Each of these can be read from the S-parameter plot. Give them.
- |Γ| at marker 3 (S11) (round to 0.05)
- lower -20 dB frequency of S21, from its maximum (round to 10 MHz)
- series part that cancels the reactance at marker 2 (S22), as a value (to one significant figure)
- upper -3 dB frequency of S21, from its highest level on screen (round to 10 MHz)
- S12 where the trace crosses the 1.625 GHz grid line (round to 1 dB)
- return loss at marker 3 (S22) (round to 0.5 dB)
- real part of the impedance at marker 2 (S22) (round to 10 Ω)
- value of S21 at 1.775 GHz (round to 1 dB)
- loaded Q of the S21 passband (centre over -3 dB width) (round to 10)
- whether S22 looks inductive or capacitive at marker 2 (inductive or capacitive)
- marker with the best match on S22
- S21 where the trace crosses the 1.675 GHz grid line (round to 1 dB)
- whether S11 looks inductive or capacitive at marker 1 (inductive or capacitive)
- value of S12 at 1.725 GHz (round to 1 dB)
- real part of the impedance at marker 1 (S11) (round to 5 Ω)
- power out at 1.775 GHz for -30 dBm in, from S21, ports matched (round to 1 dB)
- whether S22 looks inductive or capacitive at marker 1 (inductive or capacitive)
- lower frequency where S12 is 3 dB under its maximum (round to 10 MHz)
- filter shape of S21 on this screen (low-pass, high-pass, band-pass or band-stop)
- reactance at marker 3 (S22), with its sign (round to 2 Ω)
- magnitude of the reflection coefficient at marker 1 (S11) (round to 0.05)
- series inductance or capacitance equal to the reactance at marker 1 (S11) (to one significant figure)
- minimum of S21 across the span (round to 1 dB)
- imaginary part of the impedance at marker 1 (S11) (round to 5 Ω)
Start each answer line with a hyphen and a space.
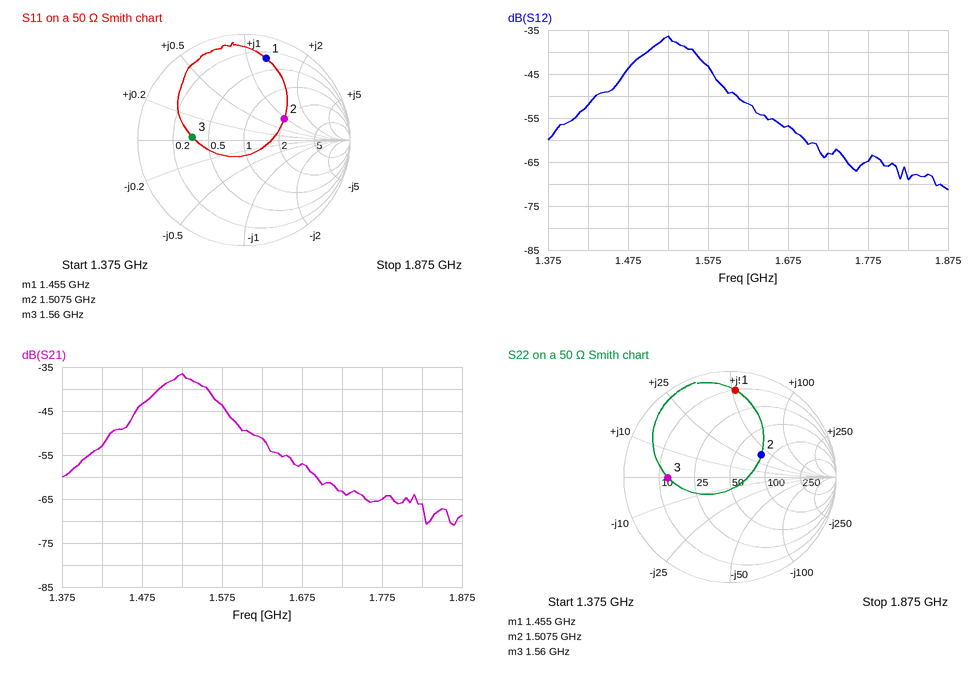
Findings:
- 0.50
- 1.40 GHz
- 3 pF
- 1.55 GHz
- -52 dB
- 4.5 dB
- 80 Ω
- -65 dB
- 30
- inductive
- marker 2
- -57 dB
- inductive
- -63 dB
- 15 Ω
- -95 dBm
- inductive
- 1.50 GHz
- band-pass
- 0 Ω
- 0.80
- 7 nH
- -71 dB
- +65 Ω
